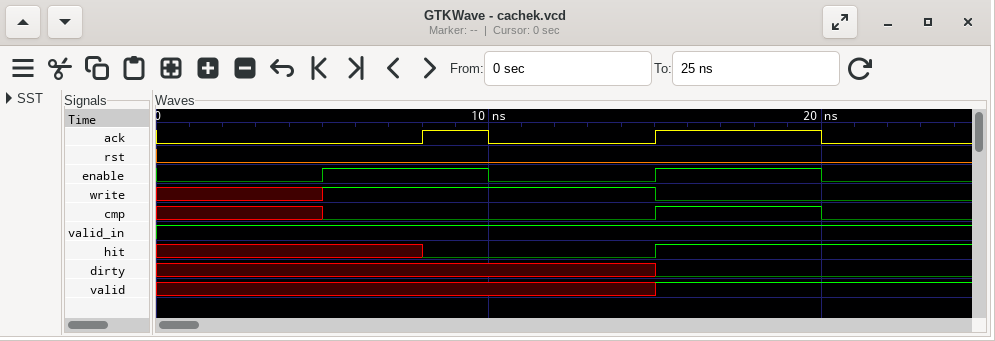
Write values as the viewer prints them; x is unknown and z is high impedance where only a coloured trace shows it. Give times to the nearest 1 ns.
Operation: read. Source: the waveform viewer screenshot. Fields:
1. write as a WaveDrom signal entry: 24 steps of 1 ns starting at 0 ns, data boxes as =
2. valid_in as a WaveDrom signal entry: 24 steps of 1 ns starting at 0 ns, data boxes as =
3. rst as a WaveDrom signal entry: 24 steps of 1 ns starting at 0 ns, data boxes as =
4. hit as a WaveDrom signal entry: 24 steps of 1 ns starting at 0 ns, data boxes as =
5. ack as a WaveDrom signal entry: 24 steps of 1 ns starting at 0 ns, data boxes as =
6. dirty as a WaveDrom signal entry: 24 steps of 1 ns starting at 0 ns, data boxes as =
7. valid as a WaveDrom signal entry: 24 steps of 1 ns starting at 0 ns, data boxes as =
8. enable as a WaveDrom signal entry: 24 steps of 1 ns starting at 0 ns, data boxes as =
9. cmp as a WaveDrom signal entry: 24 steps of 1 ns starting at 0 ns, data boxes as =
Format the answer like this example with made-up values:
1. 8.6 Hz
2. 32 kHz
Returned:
1. {name: 'write', wave: 'x....1.........0........'}
2. {name: 'valid_in', wave: '1.......................'}
3. {name: 'rst', wave: '0.......................'}
4. {name: 'hit', wave: 'x.......0......1........'}
5. {name: 'ack', wave: '0.......1.0....1....0...'}
6. {name: 'dirty', wave: 'x..............0........'}
7. {name: 'valid', wave: 'x..............1........'}
8. {name: 'enable', wave: '0....1....0....1....0...'}
9. {name: 'cmp', wave: 'x....0.........1....0...'}
